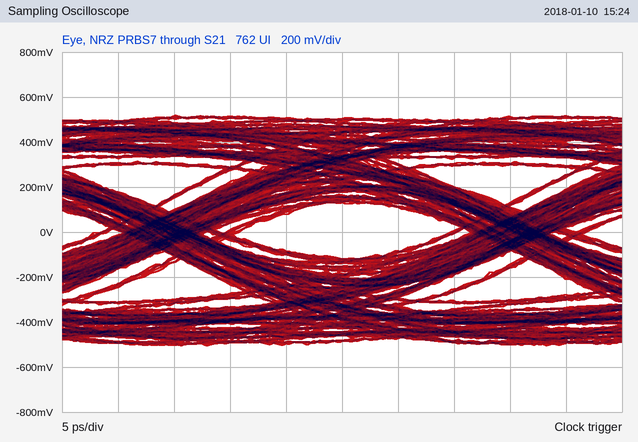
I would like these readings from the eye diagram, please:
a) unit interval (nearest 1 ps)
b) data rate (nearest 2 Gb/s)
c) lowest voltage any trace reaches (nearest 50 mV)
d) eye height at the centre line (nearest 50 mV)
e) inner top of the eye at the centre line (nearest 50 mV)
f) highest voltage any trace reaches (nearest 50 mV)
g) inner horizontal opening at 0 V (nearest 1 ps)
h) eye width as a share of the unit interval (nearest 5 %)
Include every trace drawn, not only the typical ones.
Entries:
31 ps
32 Gb/s
-500 mV
250 mV
150 mV
500 mV
19 ps
60 %
